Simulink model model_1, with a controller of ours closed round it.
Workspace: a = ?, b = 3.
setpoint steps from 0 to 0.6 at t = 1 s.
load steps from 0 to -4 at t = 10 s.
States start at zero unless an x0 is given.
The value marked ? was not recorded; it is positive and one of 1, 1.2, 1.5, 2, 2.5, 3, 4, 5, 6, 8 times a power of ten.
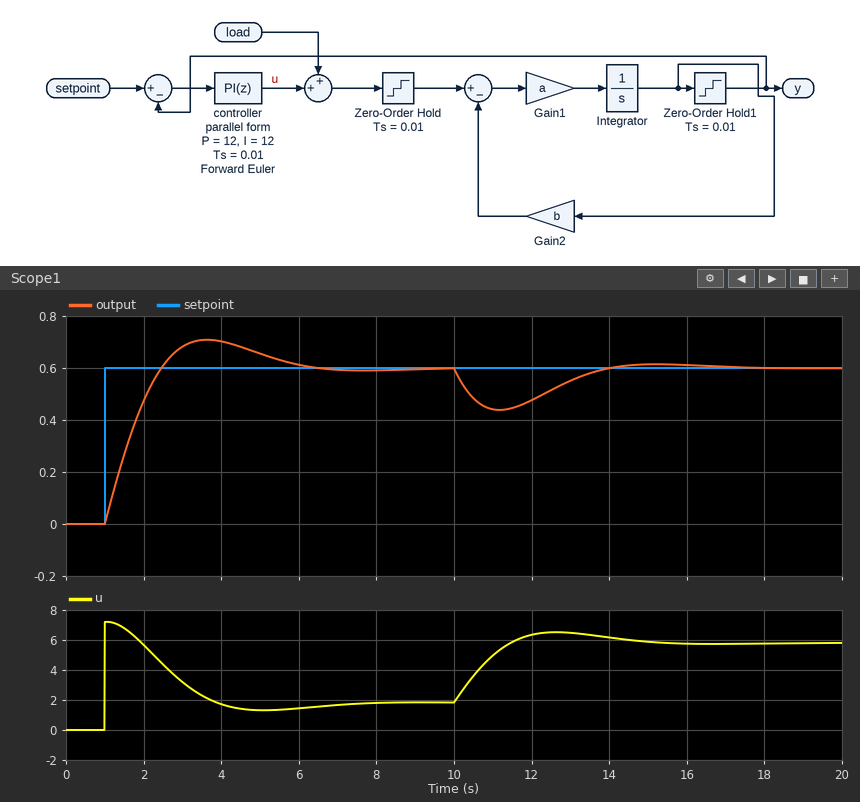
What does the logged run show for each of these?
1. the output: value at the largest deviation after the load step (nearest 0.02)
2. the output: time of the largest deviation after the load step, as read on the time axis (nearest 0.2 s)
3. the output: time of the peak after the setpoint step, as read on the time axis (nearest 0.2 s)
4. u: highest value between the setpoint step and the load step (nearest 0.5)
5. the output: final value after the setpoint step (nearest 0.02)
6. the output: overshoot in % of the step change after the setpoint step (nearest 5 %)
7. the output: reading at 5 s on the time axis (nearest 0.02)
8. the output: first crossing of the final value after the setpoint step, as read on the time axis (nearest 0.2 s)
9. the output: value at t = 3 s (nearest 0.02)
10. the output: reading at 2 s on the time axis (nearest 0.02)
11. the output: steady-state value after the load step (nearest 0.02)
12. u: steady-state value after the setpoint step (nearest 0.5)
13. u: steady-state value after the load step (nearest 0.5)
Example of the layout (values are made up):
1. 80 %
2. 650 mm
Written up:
1. 0.44
2. 11.2 s
3. 3.6 s
4. 7.0
5. 0.60
6. 20 %
7. 0.66
8. 2.4 s
9. 0.68
10. 0.48
11. 0.60
12. 2.0
13. 6.0
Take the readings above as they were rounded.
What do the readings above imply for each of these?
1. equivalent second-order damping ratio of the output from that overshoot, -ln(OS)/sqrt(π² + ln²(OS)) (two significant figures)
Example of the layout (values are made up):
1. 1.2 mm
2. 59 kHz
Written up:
1. 0.46
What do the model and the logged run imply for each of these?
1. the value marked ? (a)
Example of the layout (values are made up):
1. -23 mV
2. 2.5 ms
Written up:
1. 0.08
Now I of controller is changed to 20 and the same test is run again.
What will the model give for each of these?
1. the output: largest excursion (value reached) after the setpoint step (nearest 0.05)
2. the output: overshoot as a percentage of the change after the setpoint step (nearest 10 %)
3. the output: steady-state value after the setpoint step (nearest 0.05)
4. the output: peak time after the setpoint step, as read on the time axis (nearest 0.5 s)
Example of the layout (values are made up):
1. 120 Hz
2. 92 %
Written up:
1. 0.75
2. 30 %
3. 0.60
4. 3.0 s
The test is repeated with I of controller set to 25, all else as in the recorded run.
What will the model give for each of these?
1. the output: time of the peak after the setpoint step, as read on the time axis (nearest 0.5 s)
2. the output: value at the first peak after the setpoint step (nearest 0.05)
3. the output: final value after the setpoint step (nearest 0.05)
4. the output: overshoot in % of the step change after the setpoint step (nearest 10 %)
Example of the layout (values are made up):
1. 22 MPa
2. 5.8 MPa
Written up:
1. 3.0 s
2. 0.80
3. 0.60
4. 30 %
